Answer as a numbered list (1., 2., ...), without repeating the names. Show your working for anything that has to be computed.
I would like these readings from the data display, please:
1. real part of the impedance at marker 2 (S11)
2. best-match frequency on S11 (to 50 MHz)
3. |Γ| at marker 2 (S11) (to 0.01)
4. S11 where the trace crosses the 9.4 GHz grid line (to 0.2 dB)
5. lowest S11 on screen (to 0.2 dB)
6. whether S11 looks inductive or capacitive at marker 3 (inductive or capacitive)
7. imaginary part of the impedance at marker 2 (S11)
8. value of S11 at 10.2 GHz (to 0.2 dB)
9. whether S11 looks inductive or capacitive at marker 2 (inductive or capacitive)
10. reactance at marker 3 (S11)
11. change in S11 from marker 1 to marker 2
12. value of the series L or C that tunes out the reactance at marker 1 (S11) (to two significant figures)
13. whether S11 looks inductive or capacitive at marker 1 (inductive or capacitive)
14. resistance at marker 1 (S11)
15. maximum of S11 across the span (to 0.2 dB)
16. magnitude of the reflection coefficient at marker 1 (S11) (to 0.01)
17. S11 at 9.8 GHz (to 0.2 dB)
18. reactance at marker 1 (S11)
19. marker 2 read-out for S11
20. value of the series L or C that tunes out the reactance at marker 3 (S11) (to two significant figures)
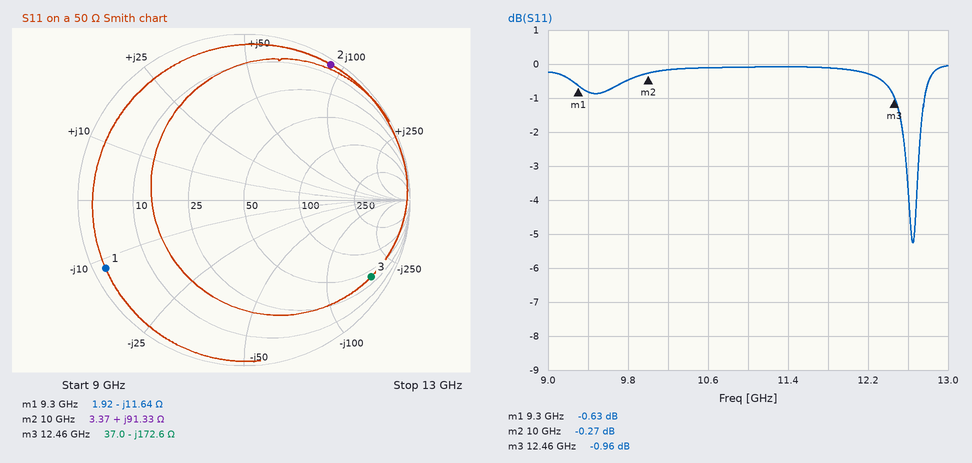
1. 3.37 Ω
2. 12.65 GHz
3. 0.97
4. -0.8 dB
5. -5.2 dB
6. capacitive
7. +91.33 Ω
8. -0.2 dB
9. inductive
10. -172.6 Ω
11. -0.27 − (-0.63) = 0.36 dB
12. L = 11.64 Ω/(2π × 9.3 GHz) ≈ 199 pH, so 200 pH to two significant figures
13. capacitive
14. 1.92 Ω
15. 0.0 dB
16. 0.93
17. -0.4 dB
18. -11.64 Ω
19. -0.27 dB
20. L = 172.6 Ω/(2π × 12.46 GHz) ≈ 2.2 nH
